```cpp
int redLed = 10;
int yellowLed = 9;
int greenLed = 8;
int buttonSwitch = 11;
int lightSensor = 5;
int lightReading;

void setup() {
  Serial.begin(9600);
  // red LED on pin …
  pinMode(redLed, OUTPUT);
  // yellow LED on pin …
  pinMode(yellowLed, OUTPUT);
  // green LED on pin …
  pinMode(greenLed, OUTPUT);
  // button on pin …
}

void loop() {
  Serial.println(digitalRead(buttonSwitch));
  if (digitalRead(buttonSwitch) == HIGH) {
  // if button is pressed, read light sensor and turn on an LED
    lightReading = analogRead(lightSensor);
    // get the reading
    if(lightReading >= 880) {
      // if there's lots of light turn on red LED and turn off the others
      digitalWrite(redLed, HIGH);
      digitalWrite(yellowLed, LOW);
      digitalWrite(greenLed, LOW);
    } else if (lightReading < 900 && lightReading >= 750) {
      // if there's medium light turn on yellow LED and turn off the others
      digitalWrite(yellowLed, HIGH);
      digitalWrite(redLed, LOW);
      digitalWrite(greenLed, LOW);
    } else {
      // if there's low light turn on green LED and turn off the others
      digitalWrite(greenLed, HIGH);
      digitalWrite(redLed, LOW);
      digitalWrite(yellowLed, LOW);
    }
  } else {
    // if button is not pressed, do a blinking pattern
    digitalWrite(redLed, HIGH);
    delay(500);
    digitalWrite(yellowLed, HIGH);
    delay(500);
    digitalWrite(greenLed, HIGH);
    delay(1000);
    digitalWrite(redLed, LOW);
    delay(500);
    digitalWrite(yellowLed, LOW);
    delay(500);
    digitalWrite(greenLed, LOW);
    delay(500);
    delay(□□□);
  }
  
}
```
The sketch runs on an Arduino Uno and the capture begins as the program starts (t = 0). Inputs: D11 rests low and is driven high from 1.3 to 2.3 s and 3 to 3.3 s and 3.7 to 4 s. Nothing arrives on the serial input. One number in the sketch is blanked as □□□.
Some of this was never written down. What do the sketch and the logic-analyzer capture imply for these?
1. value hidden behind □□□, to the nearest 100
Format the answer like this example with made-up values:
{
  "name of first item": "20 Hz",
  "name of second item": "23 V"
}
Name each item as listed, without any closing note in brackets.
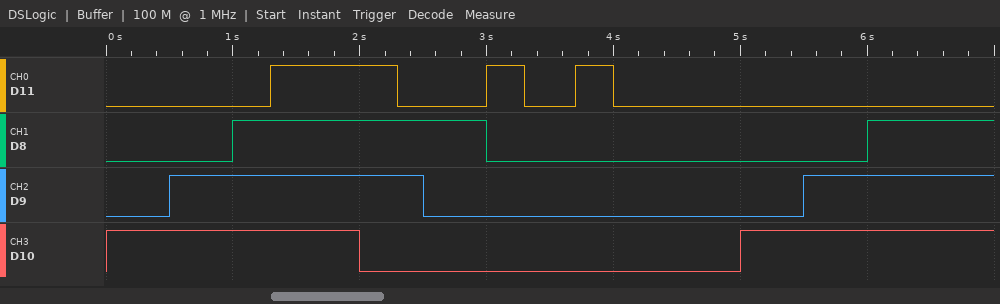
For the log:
{
  "value hidden behind □□□, to the nearest 100": "1500"
}
